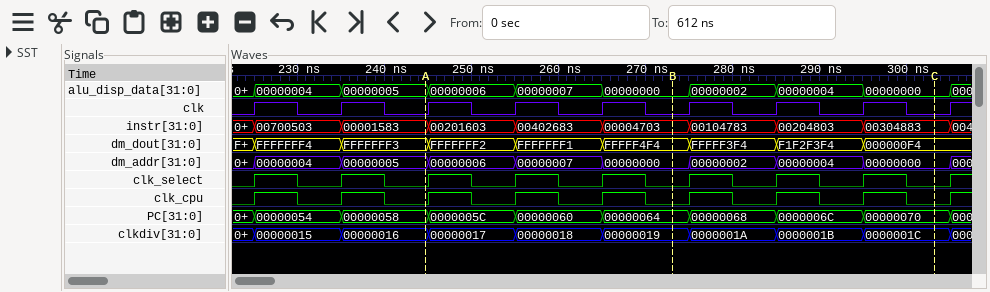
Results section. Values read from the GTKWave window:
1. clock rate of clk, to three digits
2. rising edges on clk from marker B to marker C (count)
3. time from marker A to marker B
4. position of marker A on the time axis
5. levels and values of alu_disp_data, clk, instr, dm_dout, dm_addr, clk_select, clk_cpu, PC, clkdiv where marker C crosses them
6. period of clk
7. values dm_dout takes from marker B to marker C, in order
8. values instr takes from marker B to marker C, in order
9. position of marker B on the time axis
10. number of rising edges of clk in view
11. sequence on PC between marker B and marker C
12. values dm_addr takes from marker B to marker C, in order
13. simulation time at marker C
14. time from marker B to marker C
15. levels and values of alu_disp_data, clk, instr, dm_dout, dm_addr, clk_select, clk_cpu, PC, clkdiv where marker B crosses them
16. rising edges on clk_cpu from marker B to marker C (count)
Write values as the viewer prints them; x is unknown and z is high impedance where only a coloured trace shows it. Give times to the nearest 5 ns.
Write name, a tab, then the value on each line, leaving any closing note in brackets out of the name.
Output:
clock rate of clk, to three digits	100 MHz
rising edges on clk from marker B to marker C	3
time from marker A to marker B	30 ns
position of marker A on the time axis	245 ns
levels and values of alu_disp_data, clk, instr, dm_dout, dm_addr, clk_select, clk_cpu, PC, clkdiv where marker C crosses them	alu_disp_data=00000000, clk=0, instr=00304883, dm_dout=000000F4, dm_addr=00000000, clk_select=0, clk_cpu=0, PC=00000070, clkdiv=0000001C
period of clk	10 ns
values dm_dout takes from marker B to marker C, in order	FFFFF4F4, FFFFF3F4, F1F2F3F4, 000000F4
values instr takes from marker B to marker C, in order	00004703, 00104783, 00204803, 00304883
position of marker B on the time axis	275 ns
number of rising edges of clk in view	9
sequence on PC between marker B and marker C	00000064, 00000068, 0000006C, 00000070
values dm_addr takes from marker B to marker C, in order	00000000, 00000002, 00000004, 00000000
simulation time at marker C	305 ns
time from marker B to marker C	30 ns
levels and values of alu_disp_data, clk, instr, dm_dout, dm_addr, clk_select, clk_cpu, PC, clkdiv where marker B crosses them	alu_disp_data=00000000, clk=0, instr=00004703, dm_dout=FFFFF4F4, dm_addr=00000000, clk_select=0, clk_cpu=0, PC=00000064, clkdiv=00000019
rising edges on clk_cpu from marker B to marker C	3
